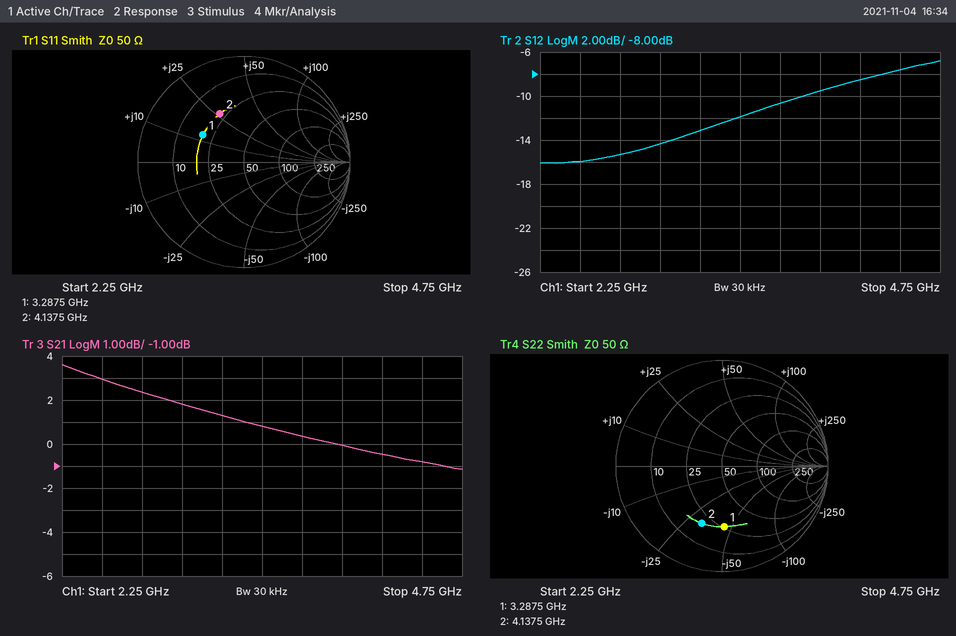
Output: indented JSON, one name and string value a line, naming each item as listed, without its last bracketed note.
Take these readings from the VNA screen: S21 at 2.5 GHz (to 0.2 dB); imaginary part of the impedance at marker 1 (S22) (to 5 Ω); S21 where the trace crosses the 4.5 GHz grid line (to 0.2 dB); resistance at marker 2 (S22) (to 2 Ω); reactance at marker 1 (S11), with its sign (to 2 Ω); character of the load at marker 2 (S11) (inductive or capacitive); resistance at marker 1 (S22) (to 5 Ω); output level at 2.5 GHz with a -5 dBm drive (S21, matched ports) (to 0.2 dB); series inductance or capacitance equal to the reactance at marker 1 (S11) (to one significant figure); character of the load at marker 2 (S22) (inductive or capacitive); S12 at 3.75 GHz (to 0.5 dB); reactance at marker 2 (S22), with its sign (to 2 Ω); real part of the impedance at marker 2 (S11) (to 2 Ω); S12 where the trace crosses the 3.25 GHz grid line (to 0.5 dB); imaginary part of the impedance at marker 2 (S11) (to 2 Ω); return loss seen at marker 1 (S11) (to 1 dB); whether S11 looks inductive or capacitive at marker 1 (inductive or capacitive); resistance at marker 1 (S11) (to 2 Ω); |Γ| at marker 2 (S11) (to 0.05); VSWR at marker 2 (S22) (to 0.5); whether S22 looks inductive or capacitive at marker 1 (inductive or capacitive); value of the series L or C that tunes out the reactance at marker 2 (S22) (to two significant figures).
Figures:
{
  "S21 at 2.5 GHz": "3.0 dB",
  "imaginary part of the impedance at marker 1 (S22)": "-45 Ω",
  "S21 where the trace crosses the 4.5 GHz grid line": "-0.8 dB",
  "resistance at marker 2 (S22)": "20 Ω",
  "reactance at marker 1 (S11), with its sign": "+12 Ω",
  "character of the load at marker 2 (S11)": "inductive",
  "resistance at marker 1 (S22)": "25 Ω",
  "output level at 2.5 GHz with a -5 dBm drive (S21, matched ports)": "-2.0 dBm",
  "series inductance or capacitance equal to the reactance at marker 1 (S11)": "600 pH",
  "character of the load at marker 2 (S22)": "capacitive",
  "S12 at 3.75 GHz": "-10.5 dB",
  "reactance at marker 2 (S22), with its sign": "-32 Ω",
  "real part of the impedance at marker 2 (S11)": "22 Ω",
  "S12 where the trace crosses the 3.25 GHz grid line": "-13.0 dB",
  "imaginary part of the impedance at marker 2 (S11)": "+26 Ω",
  "return loss seen at marker 1 (S11)": "7 dB",
  "whether S11 looks inductive or capacitive at marker 1": "inductive",
  "resistance at marker 1 (S11)": "20 Ω",
  "|Γ| at marker 2 (S11)": "0.50",
  "VSWR at marker 2 (S22)": "3.5",
  "whether S22 looks inductive or capacitive at marker 1": "capacitive",
  "value of the series L or C that tunes out the reactance at marker 2 (S22)": "1.2 nH"
}
